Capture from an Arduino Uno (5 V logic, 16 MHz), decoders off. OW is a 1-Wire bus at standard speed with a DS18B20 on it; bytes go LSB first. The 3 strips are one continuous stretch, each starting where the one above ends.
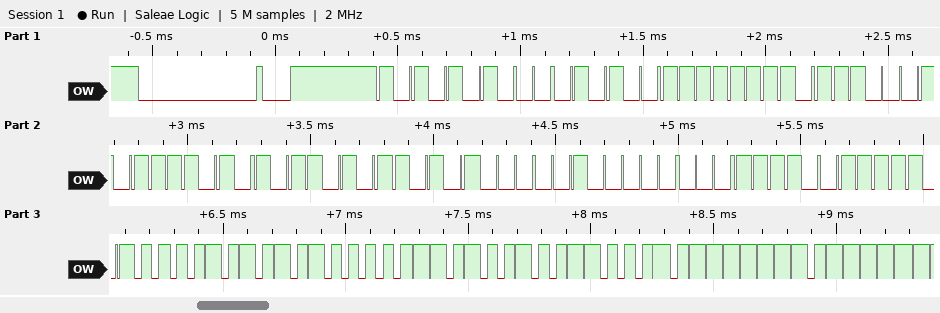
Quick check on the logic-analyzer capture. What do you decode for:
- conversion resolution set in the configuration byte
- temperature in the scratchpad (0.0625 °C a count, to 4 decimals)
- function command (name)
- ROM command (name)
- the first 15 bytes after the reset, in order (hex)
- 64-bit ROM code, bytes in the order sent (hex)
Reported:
12 bits
85.0000 °C
Read Scratchpad
Match ROM
55 28 FF 8E 5E AD 15 04 78 BE 50 05 4B 46 7F
28 FF 8E 5E AD 15 04 78
